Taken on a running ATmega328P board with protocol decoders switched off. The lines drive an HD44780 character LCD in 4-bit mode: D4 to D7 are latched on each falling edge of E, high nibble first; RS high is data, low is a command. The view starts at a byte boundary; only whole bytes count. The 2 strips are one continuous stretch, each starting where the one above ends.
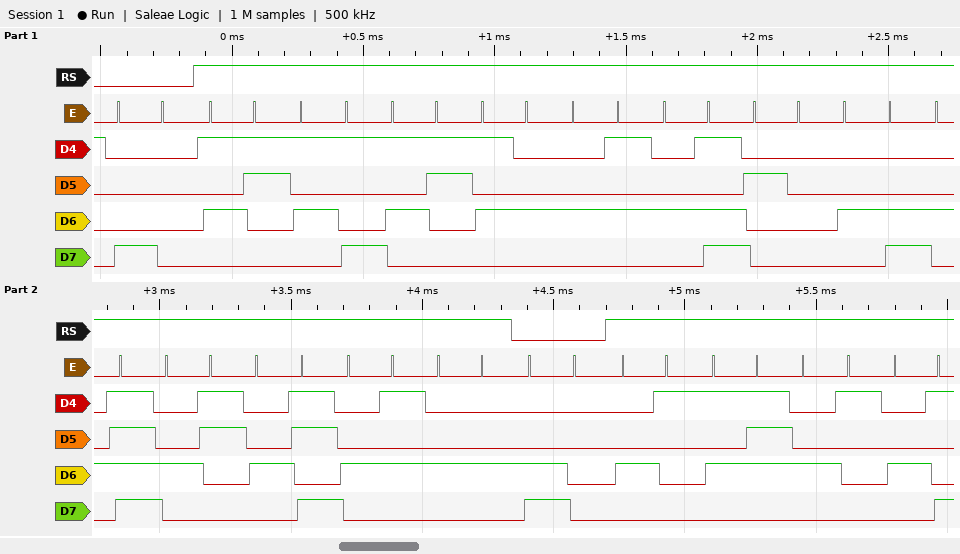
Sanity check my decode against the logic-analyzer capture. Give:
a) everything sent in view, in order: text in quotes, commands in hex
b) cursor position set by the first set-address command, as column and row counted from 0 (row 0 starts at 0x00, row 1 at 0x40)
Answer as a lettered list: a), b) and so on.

a) 0x80 "SYSTEM LOCKED" 0xC0 "AWAI"
b) column 0, row 0
